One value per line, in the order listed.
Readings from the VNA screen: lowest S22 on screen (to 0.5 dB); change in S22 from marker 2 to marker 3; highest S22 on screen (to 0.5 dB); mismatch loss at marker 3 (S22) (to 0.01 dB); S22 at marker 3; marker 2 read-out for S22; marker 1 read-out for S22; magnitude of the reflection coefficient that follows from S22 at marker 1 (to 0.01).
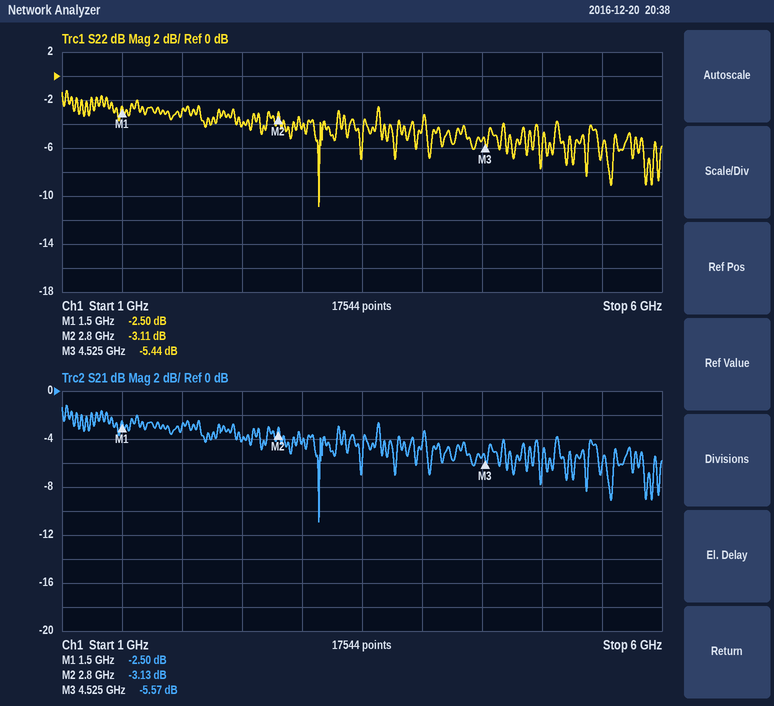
-11.0 dB
-2.33 dB
-1.0 dB
1.46 dB
-5.44 dB
-3.11 dB
-2.50 dB
0.75
